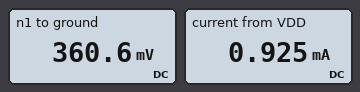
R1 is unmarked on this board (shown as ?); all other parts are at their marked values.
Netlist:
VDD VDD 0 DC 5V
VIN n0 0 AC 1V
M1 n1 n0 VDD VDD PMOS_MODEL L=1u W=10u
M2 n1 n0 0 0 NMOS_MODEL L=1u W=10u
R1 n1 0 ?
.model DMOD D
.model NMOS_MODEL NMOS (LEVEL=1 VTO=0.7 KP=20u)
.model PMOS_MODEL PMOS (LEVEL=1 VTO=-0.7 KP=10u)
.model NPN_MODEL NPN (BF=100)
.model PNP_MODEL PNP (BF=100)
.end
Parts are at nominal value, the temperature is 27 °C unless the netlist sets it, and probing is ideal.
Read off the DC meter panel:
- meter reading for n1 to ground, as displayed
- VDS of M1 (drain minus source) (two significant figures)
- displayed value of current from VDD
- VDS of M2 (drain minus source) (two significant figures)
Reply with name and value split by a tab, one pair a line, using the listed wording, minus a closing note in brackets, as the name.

meter reading for n1 to ground, as displayed	360.6 mV
VDS of M1 (drain minus source)	-4.6 V
displayed value of current from VDD	0.925 mA
VDS of M2 (drain minus source)	360 mV
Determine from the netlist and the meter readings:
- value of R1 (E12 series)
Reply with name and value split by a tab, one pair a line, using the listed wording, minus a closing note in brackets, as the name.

value of R1	390 Ω
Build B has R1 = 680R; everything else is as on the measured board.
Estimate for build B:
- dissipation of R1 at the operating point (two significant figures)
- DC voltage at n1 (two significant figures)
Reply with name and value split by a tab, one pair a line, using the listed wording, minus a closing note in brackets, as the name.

dissipation of R1 at the operating point	580 µW
DC voltage at n1	630 mV
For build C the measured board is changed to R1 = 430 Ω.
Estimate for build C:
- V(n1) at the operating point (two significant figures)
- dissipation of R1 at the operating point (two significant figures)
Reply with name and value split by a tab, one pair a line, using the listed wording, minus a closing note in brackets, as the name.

V(n1) at the operating point	400 mV
dissipation of R1 at the operating point	370 µW
